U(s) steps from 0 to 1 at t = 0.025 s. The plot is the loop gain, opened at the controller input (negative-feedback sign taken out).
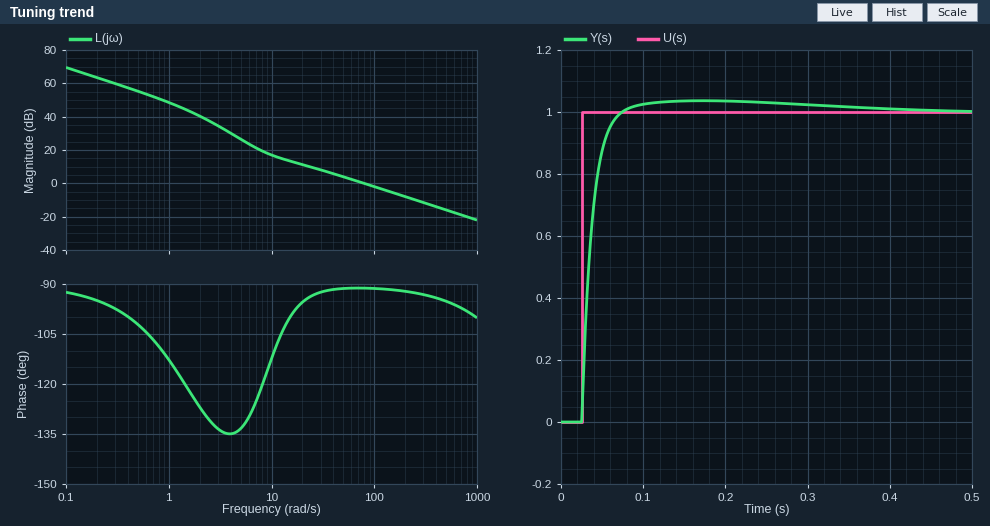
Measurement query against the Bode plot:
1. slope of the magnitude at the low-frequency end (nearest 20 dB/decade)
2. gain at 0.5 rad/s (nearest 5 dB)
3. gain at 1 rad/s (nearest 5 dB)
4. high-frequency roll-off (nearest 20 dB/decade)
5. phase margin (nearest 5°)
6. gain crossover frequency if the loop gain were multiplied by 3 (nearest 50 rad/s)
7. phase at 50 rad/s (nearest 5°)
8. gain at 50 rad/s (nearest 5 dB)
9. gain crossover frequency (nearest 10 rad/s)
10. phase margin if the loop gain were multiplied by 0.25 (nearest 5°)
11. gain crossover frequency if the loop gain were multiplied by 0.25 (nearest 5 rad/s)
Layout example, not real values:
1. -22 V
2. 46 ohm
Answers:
1. -20 dB/decade
2. 55 dB
3. 50 dB
4. -20 dB/decade
5. 90°
6. 250 rad/s
7. -90°
8. 5 dB
9. 80 rad/s
10. 85°
11. 20 rad/s
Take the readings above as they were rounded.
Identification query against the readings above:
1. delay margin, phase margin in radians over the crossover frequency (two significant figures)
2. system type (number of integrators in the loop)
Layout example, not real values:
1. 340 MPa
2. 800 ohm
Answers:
1. 0.020 s
2. 1
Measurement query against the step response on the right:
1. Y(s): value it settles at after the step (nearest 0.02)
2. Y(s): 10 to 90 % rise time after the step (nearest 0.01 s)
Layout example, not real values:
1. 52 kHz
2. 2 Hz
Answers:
1. 1.00
2. 0.03 s
